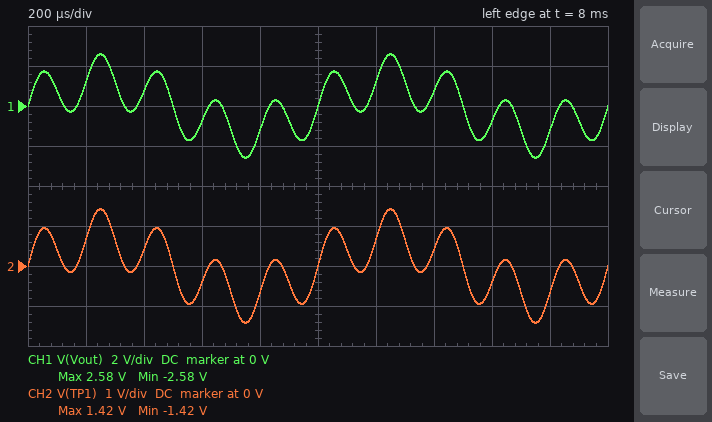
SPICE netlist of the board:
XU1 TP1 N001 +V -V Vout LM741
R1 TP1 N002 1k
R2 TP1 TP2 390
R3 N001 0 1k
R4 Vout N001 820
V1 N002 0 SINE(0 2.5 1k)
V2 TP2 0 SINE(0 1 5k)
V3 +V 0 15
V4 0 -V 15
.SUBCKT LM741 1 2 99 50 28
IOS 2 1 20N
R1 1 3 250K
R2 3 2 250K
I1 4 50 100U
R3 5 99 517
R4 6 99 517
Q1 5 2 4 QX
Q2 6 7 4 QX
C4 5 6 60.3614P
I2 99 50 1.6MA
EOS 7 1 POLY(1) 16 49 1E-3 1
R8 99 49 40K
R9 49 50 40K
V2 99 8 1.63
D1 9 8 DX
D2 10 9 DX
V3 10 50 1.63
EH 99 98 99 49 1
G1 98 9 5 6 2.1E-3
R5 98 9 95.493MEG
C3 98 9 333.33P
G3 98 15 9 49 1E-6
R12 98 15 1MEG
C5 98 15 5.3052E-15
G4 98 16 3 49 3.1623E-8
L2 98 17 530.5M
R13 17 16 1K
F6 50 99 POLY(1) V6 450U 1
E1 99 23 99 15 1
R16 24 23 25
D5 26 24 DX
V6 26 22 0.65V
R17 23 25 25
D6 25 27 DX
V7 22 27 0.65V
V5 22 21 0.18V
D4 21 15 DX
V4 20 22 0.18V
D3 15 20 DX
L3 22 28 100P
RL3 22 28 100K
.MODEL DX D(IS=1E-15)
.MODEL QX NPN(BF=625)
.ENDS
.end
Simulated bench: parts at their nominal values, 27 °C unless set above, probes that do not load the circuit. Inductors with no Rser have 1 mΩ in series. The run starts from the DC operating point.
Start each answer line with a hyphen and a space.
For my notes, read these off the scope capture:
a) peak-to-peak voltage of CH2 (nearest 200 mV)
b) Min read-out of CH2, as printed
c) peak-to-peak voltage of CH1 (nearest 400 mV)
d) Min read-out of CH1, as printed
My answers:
- 2.8 V
- -1.42 V
- 5.2 V
- -2.58 V
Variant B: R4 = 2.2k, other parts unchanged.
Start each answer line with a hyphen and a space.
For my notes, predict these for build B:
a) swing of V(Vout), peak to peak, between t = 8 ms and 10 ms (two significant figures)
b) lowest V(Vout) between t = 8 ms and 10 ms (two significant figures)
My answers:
- 9.1 V
- -4.5 V
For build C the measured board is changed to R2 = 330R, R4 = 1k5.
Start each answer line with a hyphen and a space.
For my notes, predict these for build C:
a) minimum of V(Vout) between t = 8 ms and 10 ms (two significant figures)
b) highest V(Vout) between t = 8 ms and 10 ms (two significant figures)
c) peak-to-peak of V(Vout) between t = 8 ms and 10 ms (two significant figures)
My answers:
- -3.4 V
- 3.4 V
- 6.9 V
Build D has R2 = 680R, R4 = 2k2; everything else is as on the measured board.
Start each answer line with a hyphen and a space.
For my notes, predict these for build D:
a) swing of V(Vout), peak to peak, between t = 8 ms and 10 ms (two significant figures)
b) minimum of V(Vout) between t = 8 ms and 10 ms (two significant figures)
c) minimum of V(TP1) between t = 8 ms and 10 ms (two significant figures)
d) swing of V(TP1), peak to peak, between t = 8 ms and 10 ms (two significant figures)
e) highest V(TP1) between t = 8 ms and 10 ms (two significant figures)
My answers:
- 10 V
- -5.1 V
- -1.6 V
- 3.2 V
- 1.6 V
